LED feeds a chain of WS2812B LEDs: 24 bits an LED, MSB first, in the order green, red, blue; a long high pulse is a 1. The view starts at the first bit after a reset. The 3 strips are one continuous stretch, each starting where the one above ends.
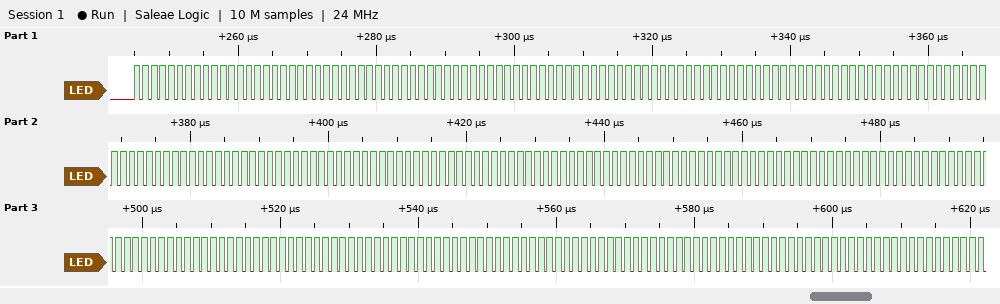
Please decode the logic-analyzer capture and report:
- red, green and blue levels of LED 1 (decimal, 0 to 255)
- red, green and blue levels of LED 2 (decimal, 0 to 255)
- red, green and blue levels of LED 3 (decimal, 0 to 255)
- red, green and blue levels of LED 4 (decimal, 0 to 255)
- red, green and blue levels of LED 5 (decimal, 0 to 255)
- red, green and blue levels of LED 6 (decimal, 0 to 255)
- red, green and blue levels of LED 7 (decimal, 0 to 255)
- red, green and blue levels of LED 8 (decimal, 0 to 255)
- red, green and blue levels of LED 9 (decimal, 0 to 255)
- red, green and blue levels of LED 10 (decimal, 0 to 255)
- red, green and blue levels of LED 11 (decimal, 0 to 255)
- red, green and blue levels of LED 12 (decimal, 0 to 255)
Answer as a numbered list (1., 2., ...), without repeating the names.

1. 255, 255, 255
2. 255, 255, 255
3. 255, 255, 255
4. 255, 255, 255
5. 255, 255, 255
6. 255, 255, 255
7. 255, 255, 255
8. 255, 255, 255
9. 255, 255, 255
10. 255, 255, 255
11. 255, 255, 255
12. 255, 255, 255
